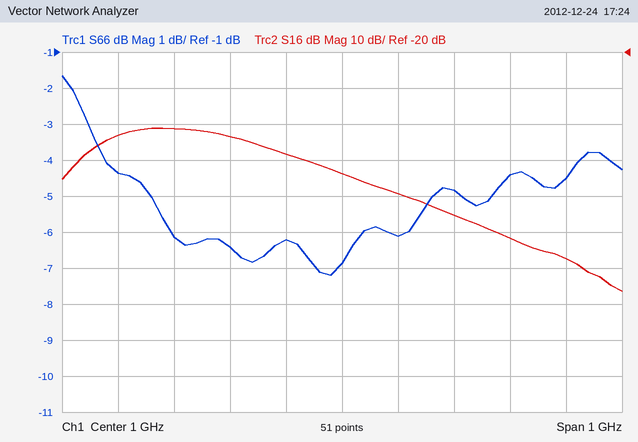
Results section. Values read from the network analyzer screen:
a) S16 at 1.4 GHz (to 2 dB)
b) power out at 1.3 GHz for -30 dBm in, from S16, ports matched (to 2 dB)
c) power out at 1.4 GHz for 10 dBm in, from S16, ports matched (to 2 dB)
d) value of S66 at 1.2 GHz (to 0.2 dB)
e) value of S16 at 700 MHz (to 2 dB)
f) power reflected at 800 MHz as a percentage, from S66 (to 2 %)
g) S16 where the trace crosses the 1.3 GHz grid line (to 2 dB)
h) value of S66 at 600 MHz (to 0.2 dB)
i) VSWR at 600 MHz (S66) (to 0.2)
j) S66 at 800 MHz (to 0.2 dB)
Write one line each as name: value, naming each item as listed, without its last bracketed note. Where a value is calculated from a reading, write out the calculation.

S16 at 1.4 GHz: -78 dB
power out at 1.3 GHz for -30 dBm in, from S16, ports matched: -30 dBm + (-72 dB) = -102 dBm
power out at 1.4 GHz for 10 dBm in, from S16, ports matched: 10 dBm + (-78 dB) = -68 dBm
value of S66 at 1.2 GHz: -4.8 dB
value of S16 at 700 MHz: -42 dB
power reflected at 800 MHz as a percentage, from S66: 10^(-6.4/10) ≈ 22.9 %, so 22 % to the nearest 2 %
S16 where the trace crosses the 1.3 GHz grid line: -72 dB
value of S66 at 600 MHz: -4.4 dB
VSWR at 600 MHz (S66): |Γ| = 10^(-4.4/20) = 0.6026; VSWR = (1 + 0.6026)/(1 − 0.6026) ≈ 4.0
S66 at 800 MHz: -6.4 dB
